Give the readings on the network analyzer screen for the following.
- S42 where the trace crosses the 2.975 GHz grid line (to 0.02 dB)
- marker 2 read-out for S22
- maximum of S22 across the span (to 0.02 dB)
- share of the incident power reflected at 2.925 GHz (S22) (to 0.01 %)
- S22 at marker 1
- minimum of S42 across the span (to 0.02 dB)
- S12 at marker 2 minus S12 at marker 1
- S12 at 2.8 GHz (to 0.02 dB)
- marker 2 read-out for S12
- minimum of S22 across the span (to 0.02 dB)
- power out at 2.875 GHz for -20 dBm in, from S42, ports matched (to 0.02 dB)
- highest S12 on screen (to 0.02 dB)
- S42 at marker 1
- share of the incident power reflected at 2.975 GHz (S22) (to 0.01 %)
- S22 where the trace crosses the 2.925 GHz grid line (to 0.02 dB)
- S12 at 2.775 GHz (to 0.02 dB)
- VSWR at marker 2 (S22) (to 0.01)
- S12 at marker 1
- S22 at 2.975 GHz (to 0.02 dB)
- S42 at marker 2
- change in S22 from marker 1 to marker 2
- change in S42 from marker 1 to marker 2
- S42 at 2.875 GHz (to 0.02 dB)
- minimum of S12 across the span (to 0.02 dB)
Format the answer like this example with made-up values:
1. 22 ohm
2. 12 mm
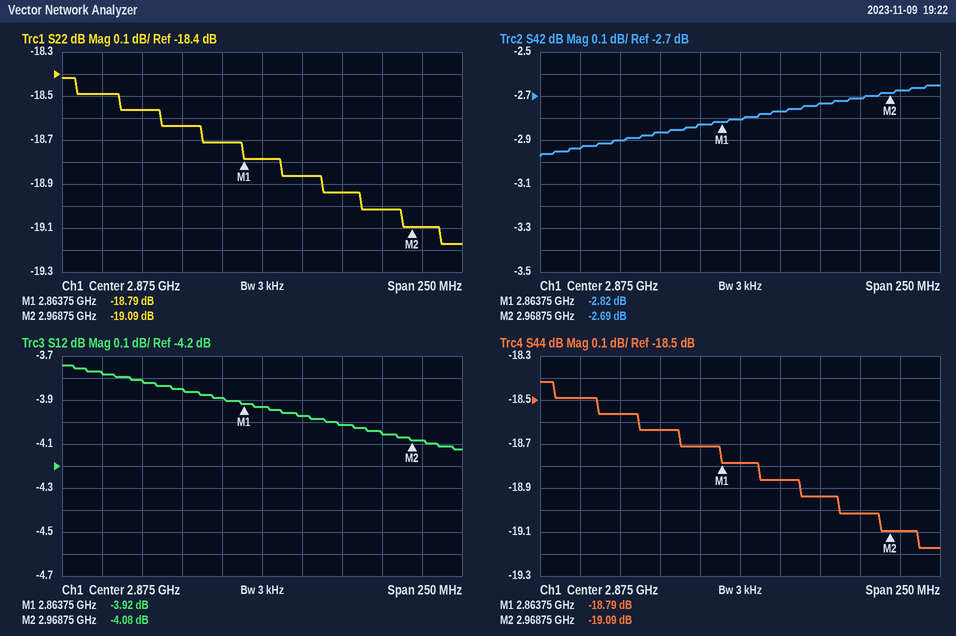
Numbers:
1. -2.68 dB
2. -19.09 dB
3. -18.42 dB
4. 1.28 %
5. -18.79 dB
6. -2.98 dB
7. -0.16 dB
8. -3.82 dB
9. -4.08 dB
10. -19.18 dB
11. -22.80 dBm
12. -3.74 dB
13. -2.82 dB
14. 1.23 %
15. -18.94 dB
16. -3.78 dB
17. 1.25
18. -3.92 dB
19. -19.10 dB
20. -2.69 dB
21. -0.30 dB
22. 0.13 dB
23. -2.80 dB
24. -4.12 dB
